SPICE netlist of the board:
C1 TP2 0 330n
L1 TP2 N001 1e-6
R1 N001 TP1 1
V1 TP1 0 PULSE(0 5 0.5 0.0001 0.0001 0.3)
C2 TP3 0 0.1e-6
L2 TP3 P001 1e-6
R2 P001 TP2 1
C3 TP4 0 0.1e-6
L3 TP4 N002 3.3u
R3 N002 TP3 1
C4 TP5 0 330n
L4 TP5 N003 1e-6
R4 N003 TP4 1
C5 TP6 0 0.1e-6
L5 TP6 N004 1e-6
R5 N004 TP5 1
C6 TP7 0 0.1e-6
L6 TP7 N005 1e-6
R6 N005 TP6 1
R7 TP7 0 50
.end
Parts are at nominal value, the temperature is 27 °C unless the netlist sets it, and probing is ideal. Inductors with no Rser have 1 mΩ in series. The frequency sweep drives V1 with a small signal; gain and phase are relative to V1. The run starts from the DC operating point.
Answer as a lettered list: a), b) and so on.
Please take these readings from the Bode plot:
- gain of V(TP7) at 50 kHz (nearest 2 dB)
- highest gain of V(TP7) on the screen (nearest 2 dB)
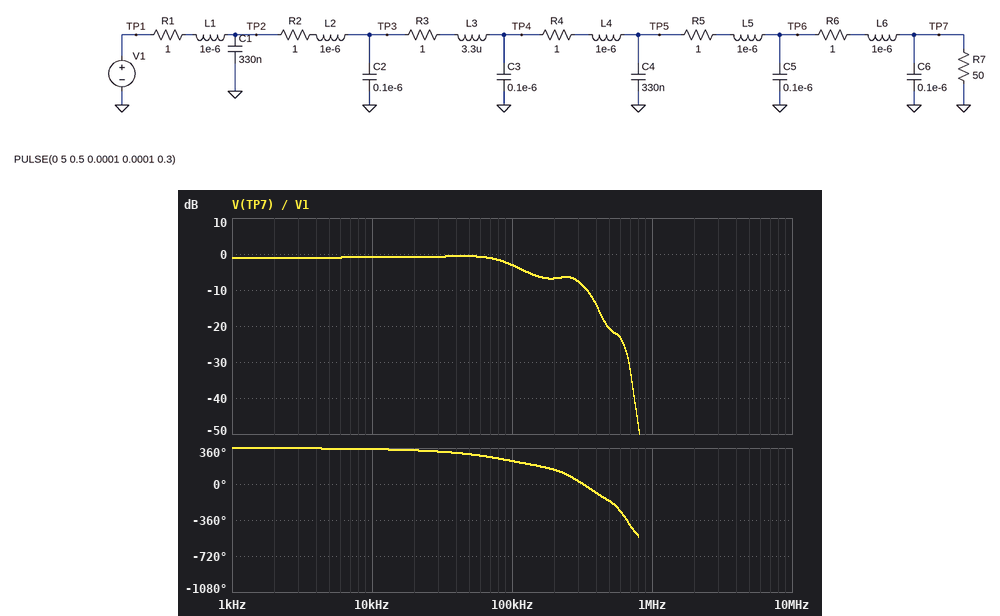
a) 0 dB
b) 0 dB
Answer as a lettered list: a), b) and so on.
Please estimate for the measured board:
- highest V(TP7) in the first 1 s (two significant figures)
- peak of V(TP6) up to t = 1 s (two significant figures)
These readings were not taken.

a) 4.5 V
b) 4.6 V
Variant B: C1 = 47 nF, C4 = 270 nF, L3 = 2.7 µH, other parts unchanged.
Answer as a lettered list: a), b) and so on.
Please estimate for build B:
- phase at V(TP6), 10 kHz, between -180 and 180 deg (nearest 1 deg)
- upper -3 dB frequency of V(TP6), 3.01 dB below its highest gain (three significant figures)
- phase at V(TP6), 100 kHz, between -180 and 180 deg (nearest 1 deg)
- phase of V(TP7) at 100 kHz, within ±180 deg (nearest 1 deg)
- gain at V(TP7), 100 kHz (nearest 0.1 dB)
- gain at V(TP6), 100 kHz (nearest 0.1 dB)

a) -9 deg
b) 110 kHz
c) -108 deg
d) -113 deg
e) -2.6 dB
f) -2.7 dB
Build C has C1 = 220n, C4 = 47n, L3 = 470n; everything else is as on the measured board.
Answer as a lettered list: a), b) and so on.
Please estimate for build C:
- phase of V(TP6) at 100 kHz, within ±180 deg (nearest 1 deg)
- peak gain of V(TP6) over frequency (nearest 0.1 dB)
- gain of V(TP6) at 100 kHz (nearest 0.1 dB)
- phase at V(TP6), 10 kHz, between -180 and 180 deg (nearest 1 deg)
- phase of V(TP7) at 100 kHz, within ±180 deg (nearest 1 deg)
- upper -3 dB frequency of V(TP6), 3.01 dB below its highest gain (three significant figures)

a) -75 deg
b) -0.3 dB
c) -0.4 dB
d) -7 deg
e) -80 deg
f) 197 kHz
